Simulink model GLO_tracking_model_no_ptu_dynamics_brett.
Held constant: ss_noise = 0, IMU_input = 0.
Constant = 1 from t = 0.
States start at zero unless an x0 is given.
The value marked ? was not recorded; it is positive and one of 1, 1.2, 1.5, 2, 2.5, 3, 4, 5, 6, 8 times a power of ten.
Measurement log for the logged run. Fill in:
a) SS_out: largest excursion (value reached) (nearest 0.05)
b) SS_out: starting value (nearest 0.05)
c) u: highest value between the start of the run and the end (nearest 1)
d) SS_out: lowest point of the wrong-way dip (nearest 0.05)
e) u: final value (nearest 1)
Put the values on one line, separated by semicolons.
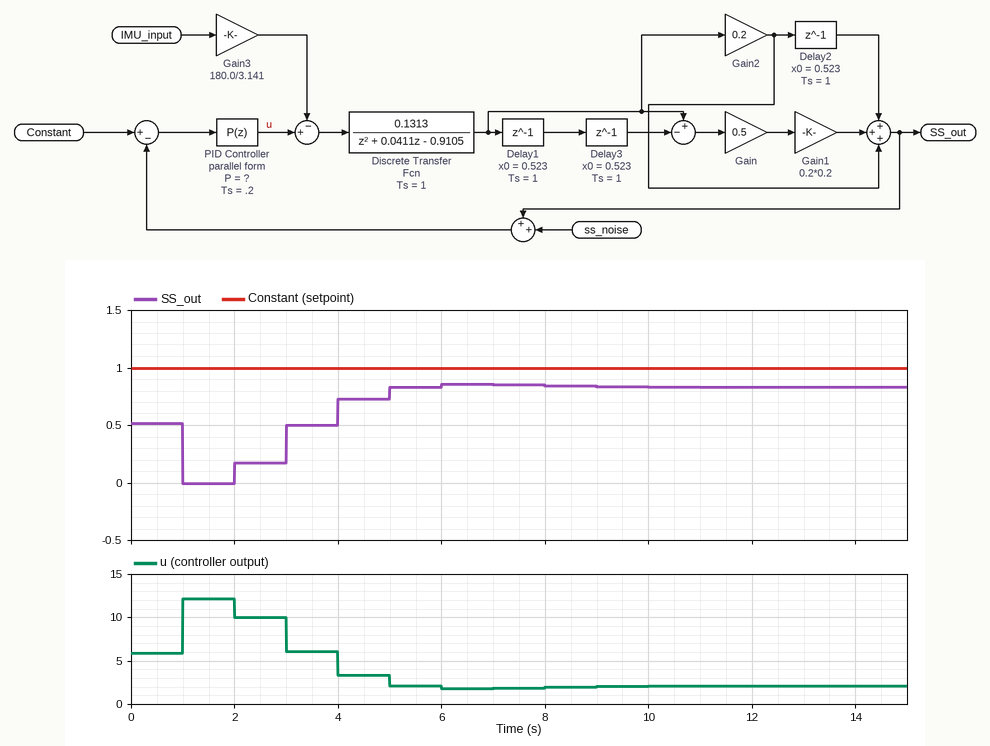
0.85; 0.50; 12; 0.00; 2
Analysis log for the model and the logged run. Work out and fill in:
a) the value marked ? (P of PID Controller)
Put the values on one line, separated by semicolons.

12
